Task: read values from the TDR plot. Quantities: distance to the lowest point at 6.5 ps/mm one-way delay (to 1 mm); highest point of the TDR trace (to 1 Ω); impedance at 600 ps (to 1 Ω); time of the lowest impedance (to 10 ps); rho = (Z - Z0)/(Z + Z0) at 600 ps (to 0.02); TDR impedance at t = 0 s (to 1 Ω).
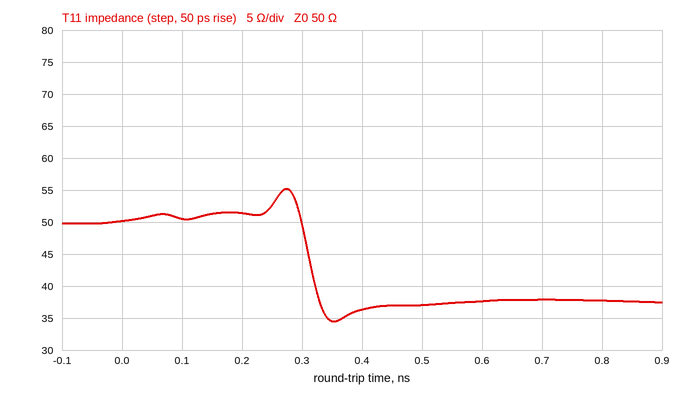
27 mm
55 Ω
38 Ω
350 ps
-0.14
50 Ω
